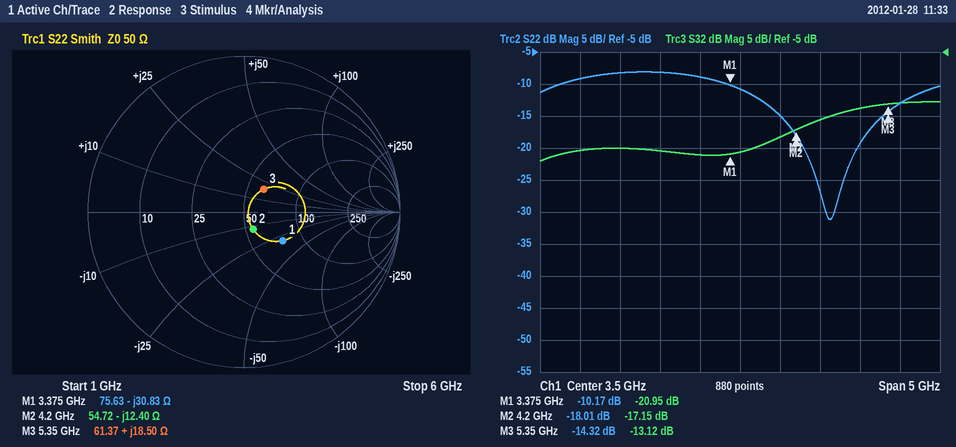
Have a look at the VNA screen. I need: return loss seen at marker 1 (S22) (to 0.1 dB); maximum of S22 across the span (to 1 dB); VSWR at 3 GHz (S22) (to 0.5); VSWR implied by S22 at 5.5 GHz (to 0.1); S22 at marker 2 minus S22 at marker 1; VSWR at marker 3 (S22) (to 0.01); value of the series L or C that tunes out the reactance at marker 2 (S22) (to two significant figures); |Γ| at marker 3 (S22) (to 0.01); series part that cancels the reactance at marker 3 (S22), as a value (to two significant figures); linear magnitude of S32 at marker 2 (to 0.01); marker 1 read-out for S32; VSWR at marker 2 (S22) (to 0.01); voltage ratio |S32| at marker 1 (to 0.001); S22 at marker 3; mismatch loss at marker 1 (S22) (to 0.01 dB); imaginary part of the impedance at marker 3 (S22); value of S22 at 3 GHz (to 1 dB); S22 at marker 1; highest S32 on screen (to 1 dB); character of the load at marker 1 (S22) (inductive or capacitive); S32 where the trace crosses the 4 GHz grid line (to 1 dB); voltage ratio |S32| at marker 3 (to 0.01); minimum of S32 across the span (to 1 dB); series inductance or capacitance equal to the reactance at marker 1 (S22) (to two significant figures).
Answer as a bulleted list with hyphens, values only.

- 10.2 dB
- -8 dB
- 2.0
- 1.6
- -7.84 dB
- 1.48
- 470 pH
- 0.19
- 1.6 pF
- 0.14
- -20.95 dB
- 1.29
- 0.090
- -14.32 dB
- 0.44 dB
- +18.50 Ω
- -9 dB
- -10.17 dB
- -13 dB
- capacitive
- -18 dB
- 0.22
- -22 dB
- 1.5 pF
